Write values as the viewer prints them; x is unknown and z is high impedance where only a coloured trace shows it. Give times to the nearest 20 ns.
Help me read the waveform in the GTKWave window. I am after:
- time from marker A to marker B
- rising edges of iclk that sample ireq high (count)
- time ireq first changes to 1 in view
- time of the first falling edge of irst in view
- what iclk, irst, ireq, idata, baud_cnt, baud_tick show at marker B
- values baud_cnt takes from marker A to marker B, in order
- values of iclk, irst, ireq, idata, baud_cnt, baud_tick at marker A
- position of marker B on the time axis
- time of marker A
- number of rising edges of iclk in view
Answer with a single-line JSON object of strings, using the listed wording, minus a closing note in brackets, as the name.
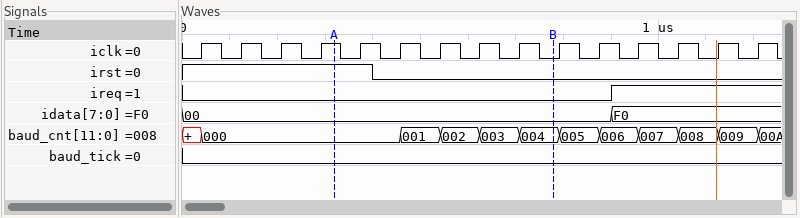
{"time from marker A to marker B": "460 ns", "rising edges of iclk that sample ireq high": "4", "time ireq first changes to 1 in view": "900 ns", "time of the first falling edge of irst in view": "400 ns", "what iclk, irst, ireq, idata, baud_cnt, baud_tick show at marker B": "iclk=0, irst=0, ireq=0, idata=00, baud_cnt=004, baud_tick=0", "values baud_cnt takes from marker A to marker B, in order": "000, 001, 002, 003, 004", "values of iclk, irst, ireq, idata, baud_cnt, baud_tick at marker A": "iclk=1, irst=1, ireq=0, idata=00, baud_cnt=000, baud_tick=0", "position of marker B on the time axis": "780 ns", "time of marker A": "320 ns", "number of rising edges of iclk in view": "15"}
